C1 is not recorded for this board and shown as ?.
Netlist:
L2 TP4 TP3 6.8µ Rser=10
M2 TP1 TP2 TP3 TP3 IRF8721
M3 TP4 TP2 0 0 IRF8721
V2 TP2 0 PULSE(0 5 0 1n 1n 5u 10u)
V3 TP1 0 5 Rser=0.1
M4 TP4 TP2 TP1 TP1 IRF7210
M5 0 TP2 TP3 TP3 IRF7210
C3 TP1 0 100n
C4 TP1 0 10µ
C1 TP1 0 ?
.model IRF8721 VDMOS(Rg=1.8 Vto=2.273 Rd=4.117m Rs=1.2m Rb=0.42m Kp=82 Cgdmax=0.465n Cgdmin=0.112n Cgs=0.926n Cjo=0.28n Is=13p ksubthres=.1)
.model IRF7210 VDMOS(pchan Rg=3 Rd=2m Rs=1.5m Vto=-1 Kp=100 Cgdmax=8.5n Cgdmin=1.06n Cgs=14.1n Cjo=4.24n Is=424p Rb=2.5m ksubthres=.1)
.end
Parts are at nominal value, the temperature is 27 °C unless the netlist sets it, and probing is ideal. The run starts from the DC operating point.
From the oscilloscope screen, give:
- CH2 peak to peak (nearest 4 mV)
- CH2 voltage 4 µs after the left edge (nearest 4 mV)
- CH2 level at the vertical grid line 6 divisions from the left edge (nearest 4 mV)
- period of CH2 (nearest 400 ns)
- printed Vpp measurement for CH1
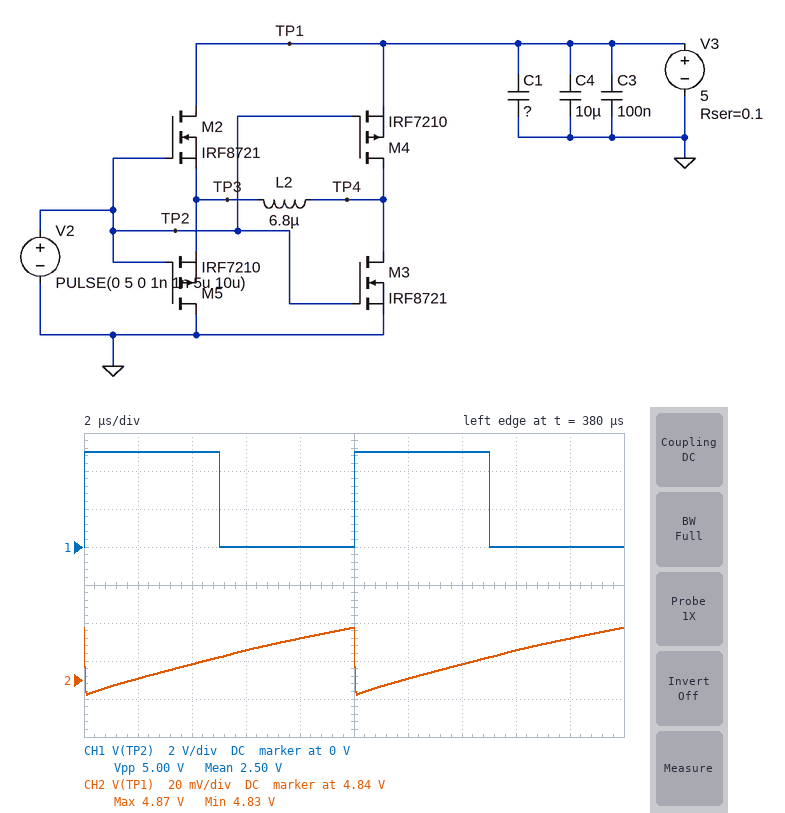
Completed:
36 mV
4.848 V
4.840 V
10.0 µs
5.00 V
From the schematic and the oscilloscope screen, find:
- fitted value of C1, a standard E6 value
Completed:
330 µF
